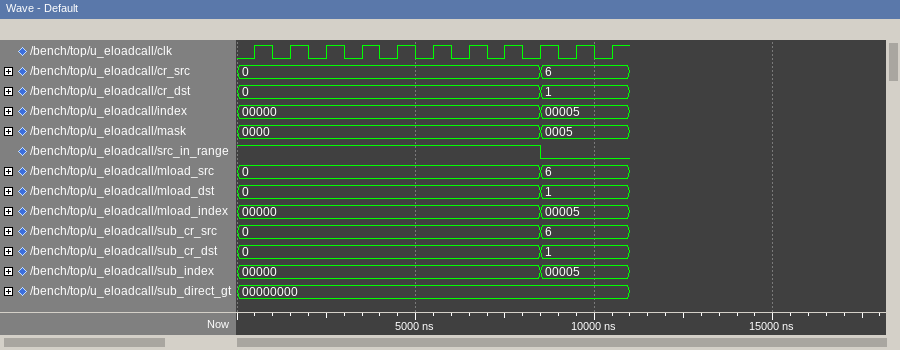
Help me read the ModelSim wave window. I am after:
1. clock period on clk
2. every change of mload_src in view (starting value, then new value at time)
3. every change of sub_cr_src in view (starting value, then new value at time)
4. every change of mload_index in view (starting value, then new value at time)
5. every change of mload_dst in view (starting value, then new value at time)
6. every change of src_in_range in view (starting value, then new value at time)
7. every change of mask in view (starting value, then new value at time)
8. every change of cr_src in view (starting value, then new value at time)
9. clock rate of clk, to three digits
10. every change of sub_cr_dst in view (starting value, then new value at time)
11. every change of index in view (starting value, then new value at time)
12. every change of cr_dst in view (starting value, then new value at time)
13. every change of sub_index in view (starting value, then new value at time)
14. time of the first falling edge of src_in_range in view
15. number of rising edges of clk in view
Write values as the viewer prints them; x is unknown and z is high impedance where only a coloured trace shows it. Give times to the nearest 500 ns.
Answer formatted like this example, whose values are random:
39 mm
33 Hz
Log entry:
1000 ns
0, 6 at 8500 ns
0, 6 at 8500 ns
00000, 00005 at 8500 ns
0, 1 at 8500 ns
1, 0 at 8500 ns
0000, 0005 at 8500 ns
0, 6 at 8500 ns
1.00 MHz
0, 1 at 8500 ns
00000, 00005 at 8500 ns
0, 1 at 8500 ns
00000, 00005 at 8500 ns
8500 ns
11
